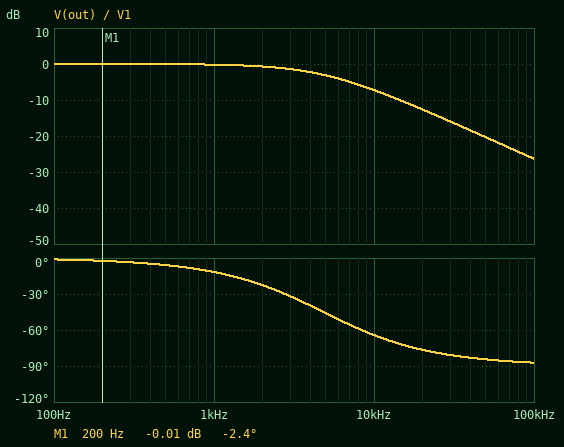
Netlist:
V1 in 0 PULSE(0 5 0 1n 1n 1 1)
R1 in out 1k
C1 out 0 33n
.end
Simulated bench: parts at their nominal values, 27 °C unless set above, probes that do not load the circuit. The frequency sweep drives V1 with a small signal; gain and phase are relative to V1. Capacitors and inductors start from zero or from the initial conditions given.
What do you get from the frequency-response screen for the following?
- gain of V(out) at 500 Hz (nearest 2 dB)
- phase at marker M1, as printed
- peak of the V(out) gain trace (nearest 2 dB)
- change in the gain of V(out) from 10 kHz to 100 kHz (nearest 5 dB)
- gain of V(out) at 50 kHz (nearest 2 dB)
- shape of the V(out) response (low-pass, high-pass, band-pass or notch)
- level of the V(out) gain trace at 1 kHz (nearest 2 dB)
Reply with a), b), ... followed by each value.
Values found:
a) 0 dB
b) -2.4 deg
c) 0 dB
d) -20 dB
e) -20 dB
f) low-pass
g) 0 dB
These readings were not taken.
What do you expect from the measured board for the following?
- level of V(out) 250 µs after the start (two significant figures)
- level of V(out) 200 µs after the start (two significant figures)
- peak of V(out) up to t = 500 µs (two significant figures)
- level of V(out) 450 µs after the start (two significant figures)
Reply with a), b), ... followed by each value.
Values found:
a) 5.0 V
b) 5.0 V
c) 5.0 V
d) 5.0 V
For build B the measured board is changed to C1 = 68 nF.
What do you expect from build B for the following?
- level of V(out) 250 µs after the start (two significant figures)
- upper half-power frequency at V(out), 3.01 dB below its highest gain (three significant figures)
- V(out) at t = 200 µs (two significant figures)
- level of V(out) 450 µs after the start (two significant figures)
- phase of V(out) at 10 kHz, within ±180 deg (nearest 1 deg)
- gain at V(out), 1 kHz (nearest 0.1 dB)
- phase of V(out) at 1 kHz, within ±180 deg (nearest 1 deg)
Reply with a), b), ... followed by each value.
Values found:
a) 4.9 V
b) 2.34 kHz
c) 4.7 V
d) 5.0 V
e) -77 deg
f) -0.7 dB
g) -23 deg
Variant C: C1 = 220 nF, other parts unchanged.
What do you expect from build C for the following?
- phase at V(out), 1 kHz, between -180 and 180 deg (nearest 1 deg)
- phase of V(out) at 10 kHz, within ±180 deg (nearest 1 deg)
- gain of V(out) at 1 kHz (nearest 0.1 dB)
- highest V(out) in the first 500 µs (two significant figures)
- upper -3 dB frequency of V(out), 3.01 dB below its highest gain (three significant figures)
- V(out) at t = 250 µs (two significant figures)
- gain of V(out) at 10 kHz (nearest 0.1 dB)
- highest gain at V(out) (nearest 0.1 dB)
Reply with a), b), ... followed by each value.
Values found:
a) -54 deg
b) -86 deg
c) -4.6 dB
d) 4.5 V
e) 723 Hz
f) 3.4 V
g) -22.8 dB
h) 0 dB
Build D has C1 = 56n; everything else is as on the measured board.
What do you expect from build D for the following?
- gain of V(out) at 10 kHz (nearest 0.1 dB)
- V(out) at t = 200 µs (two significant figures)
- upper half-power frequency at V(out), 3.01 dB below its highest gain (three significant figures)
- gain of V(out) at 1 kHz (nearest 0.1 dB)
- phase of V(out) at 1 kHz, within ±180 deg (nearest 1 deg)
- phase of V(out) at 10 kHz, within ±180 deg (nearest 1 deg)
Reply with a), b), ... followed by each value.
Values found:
a) -11.3 dB
b) 4.9 V
c) 2.84 kHz
d) -0.5 dB
e) -19 deg
f) -74 deg
